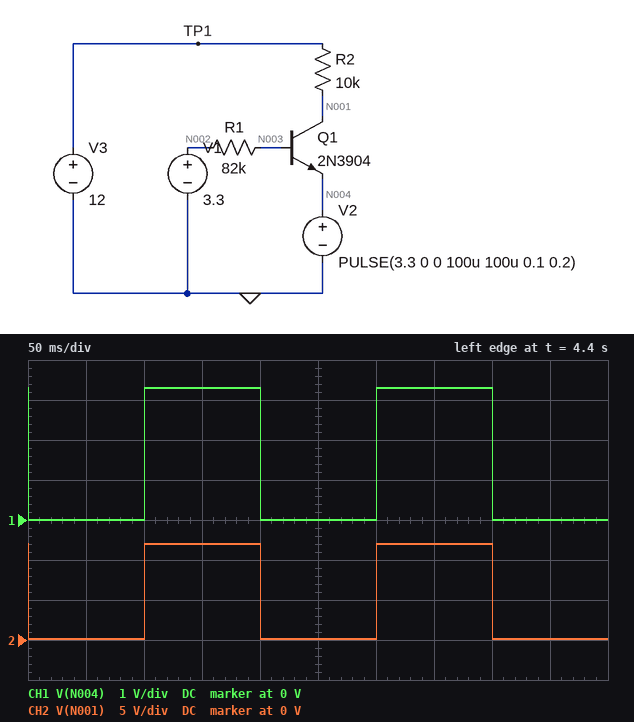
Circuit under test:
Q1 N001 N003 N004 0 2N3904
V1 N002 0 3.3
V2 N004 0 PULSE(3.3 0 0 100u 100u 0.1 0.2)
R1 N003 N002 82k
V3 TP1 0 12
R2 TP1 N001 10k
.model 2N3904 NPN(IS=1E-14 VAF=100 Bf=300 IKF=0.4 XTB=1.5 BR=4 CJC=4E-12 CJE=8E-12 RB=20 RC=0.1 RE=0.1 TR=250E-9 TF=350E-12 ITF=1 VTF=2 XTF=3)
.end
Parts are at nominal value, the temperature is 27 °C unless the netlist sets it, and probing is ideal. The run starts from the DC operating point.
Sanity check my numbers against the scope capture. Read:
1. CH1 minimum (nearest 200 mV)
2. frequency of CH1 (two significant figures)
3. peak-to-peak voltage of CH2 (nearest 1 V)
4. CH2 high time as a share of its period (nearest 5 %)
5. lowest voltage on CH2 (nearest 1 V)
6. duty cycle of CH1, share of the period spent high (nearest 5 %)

0 V
5.0 Hz
12 V
50 %
0 V
50 %
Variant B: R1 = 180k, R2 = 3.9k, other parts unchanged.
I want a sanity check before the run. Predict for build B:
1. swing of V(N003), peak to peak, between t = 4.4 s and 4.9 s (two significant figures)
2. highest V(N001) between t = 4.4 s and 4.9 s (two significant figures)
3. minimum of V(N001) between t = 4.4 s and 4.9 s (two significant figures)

2.7 V
12 V
140 mV
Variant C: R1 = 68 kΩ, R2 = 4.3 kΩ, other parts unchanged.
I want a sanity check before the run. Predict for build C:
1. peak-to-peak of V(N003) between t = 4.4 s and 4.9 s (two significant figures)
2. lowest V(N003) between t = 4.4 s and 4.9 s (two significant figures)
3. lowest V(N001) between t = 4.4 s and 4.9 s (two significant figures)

2.7 V
680 mV
85 mV
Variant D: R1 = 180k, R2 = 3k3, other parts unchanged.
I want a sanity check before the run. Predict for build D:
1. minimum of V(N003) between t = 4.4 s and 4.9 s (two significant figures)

690 mV
